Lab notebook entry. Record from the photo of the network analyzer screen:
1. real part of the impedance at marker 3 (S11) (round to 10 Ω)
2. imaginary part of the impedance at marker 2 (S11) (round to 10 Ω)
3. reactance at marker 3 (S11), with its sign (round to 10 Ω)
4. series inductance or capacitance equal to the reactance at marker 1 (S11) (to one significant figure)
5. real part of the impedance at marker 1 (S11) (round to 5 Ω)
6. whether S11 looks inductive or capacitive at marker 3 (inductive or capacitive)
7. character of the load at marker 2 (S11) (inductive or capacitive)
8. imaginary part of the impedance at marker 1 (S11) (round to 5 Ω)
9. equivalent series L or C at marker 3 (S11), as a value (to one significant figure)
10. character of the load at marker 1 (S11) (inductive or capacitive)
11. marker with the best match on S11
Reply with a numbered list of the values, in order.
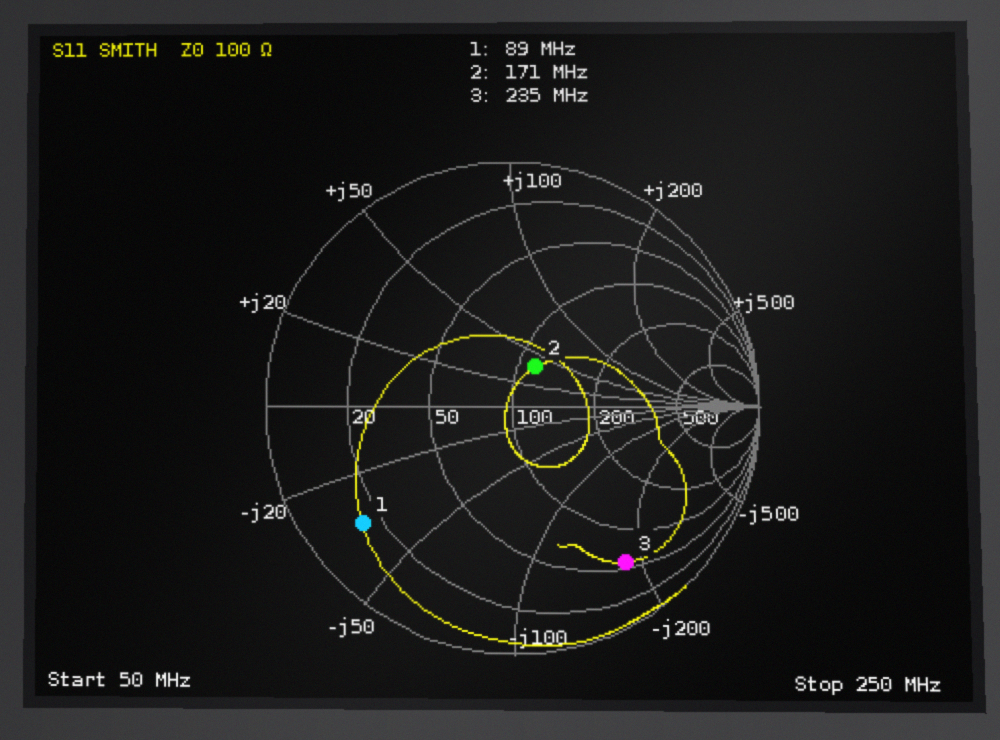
1. 60 Ω
2. +40 Ω
3. -180 Ω
4. 50 pF
5. 15 Ω
6. capacitive
7. inductive
8. -35 Ω
9. 4 pF
10. capacitive
11. marker 2
